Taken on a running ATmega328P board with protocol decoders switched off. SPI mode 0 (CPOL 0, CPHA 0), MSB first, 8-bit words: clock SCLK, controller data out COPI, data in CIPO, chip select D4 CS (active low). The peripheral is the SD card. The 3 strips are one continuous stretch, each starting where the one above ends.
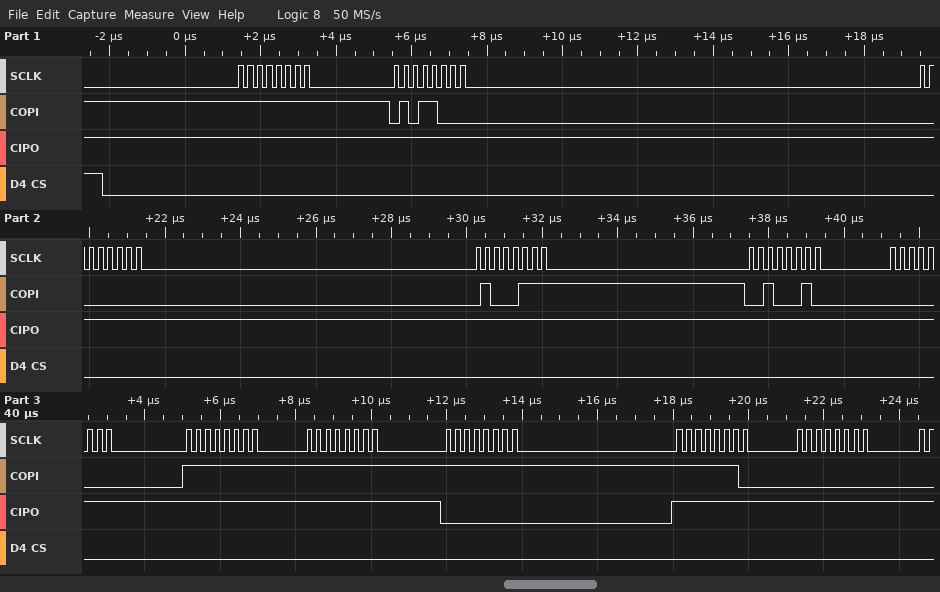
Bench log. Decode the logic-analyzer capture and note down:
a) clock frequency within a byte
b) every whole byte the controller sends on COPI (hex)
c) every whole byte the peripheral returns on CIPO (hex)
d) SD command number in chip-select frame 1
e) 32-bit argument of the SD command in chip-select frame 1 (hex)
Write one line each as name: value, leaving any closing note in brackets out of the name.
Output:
clock frequency within a byte: 4 MHz
every whole byte the controller sends on COPI: 0xFF 0x58 0x00 0x47 0x22 0x00 0xFF 0xFF 0xFF 0xFE 0x00
every whole byte the peripheral returns on CIPO: 0xFF 0xFF 0xFF 0xFF 0xFF 0xFF 0xFF 0xFF 0x00 0xFF 0xFF
SD command number in chip-select frame 1: CMD24
32-bit argument of the SD command in chip-select frame 1: 0x00472200
